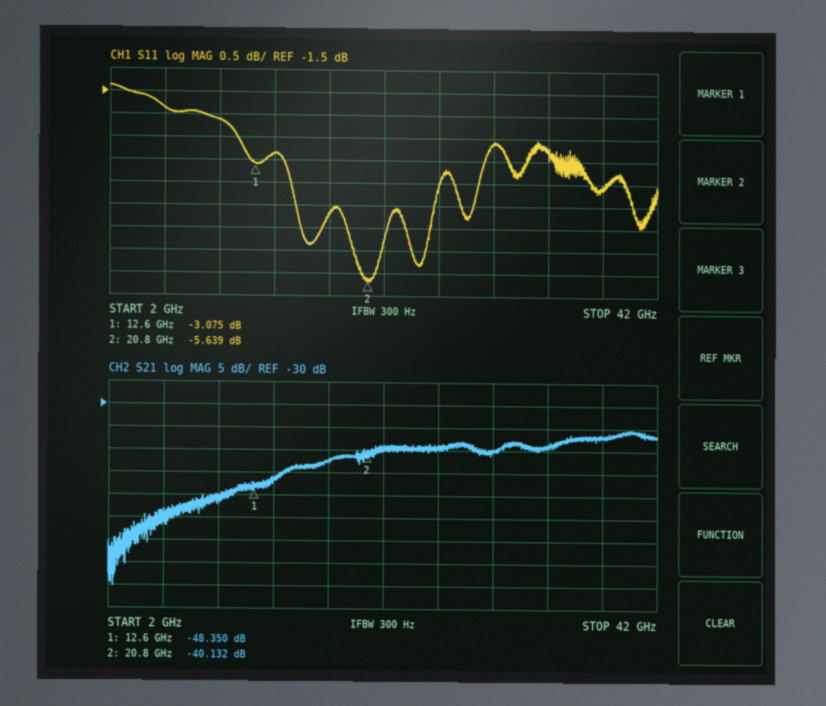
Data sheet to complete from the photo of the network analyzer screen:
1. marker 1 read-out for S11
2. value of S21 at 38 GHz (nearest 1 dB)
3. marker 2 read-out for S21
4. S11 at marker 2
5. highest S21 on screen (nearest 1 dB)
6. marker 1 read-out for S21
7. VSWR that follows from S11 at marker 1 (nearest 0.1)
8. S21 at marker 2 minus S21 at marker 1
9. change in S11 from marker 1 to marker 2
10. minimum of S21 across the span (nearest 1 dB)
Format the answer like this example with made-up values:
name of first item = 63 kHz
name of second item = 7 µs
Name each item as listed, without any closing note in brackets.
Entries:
marker 1 read-out for S11 = -3.075 dB
value of S21 at 38 GHz = -37 dB
marker 2 read-out for S21 = -40.132 dB
S11 at marker 2 = -5.639 dB
highest S21 on screen = -35 dB
marker 1 read-out for S21 = -48.350 dB
VSWR that follows from S11 at marker 1 = 5.7
S21 at marker 2 minus S21 at marker 1 = 8.218 dB
change in S11 from marker 1 to marker 2 = -2.564 dB
minimum of S21 across the span = -70 dB
